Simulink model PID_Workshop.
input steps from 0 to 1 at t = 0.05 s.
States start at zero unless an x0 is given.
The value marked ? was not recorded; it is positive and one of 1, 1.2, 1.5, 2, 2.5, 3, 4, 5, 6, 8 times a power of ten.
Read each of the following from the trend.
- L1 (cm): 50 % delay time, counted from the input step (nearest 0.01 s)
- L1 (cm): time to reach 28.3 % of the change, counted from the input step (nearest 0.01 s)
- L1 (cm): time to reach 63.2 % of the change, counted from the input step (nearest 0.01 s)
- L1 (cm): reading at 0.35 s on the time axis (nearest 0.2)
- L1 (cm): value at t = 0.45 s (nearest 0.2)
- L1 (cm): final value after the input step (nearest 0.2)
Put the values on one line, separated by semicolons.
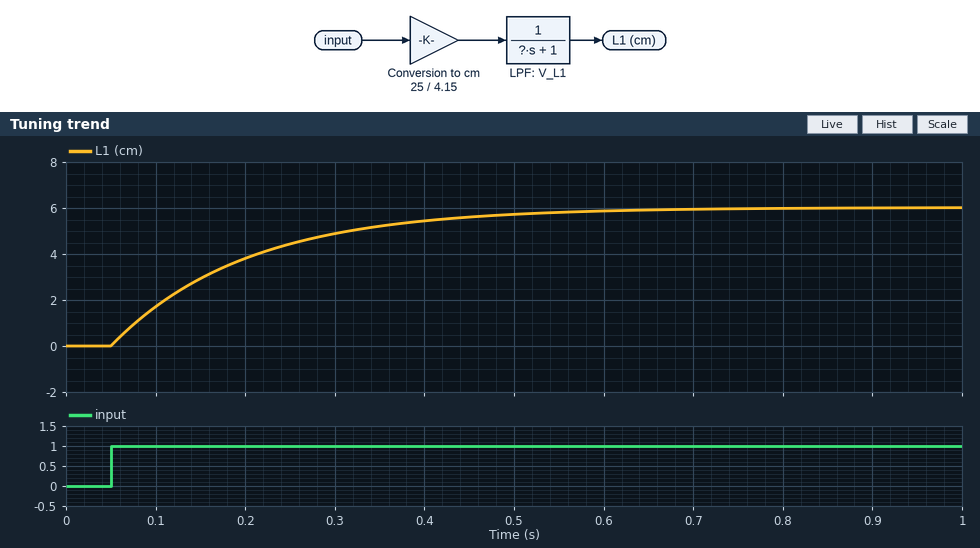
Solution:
0.10 s; 0.05 s; 0.15 s; 5.2; 5.6; 6.0
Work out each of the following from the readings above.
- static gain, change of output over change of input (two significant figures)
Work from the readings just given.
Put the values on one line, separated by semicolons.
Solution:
6.0
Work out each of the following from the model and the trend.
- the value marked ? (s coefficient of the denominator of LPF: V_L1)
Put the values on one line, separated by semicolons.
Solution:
0.15
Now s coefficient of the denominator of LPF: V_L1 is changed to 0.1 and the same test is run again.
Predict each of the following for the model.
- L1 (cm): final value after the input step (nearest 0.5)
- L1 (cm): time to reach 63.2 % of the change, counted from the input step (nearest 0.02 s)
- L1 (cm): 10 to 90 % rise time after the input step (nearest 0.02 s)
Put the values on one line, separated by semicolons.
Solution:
6.0; 0.10 s; 0.22 s
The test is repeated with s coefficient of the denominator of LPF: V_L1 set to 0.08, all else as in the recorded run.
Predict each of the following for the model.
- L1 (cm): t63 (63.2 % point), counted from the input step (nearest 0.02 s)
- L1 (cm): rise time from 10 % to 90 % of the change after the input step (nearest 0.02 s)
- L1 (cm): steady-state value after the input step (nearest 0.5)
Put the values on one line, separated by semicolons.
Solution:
0.08 s; 0.18 s; 6.0
